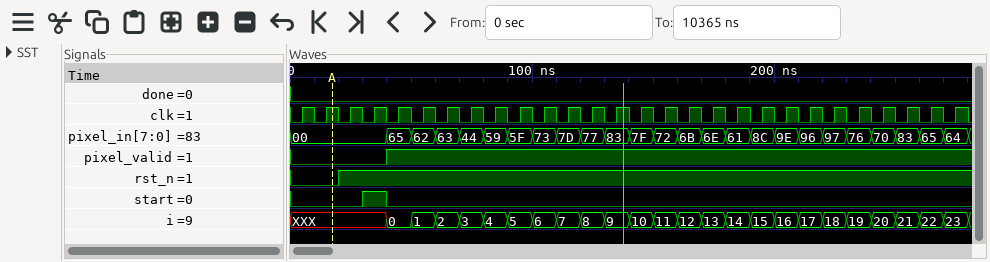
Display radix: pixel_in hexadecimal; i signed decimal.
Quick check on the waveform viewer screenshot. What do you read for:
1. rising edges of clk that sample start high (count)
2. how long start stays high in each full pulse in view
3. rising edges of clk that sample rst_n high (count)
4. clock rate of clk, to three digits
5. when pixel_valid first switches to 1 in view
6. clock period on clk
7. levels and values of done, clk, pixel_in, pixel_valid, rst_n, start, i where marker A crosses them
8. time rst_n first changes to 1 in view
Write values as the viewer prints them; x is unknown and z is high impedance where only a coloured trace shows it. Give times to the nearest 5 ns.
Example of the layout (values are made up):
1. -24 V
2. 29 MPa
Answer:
1. 1
2. 10 ns
3. 26
4. 100 MHz
5. 40 ns
6. 10 ns
7. done=0, clk=1, pixel_in=00, pixel_valid=0, rst_n=0, start=0, i=XXX
8. 20 ns
